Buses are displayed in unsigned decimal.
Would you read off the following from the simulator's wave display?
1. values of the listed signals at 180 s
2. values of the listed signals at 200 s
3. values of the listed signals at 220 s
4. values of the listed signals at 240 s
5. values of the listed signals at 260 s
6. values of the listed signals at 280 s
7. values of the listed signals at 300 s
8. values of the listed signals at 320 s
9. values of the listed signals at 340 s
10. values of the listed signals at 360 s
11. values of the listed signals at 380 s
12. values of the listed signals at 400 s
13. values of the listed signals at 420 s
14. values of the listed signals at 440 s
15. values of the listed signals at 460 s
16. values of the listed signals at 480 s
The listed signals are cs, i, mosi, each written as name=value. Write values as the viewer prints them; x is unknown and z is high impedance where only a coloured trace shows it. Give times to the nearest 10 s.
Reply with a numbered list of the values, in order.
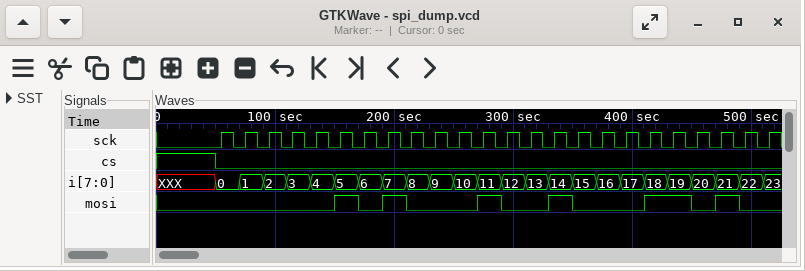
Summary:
1. cs=0, i=6, mosi=0
2. cs=0, i=7, mosi=1
3. cs=0, i=8, mosi=0
4. cs=0, i=9, mosi=0
5. cs=0, i=10, mosi=0
6. cs=0, i=11, mosi=1
7. cs=0, i=12, mosi=0
8. cs=0, i=13, mosi=0
9. cs=0, i=14, mosi=1
10. cs=0, i=15, mosi=0
11. cs=0, i=16, mosi=0
12. cs=0, i=17, mosi=0
13. cs=0, i=18, mosi=1
14. cs=0, i=19, mosi=1
15. cs=0, i=20, mosi=0
16. cs=0, i=21, mosi=1
